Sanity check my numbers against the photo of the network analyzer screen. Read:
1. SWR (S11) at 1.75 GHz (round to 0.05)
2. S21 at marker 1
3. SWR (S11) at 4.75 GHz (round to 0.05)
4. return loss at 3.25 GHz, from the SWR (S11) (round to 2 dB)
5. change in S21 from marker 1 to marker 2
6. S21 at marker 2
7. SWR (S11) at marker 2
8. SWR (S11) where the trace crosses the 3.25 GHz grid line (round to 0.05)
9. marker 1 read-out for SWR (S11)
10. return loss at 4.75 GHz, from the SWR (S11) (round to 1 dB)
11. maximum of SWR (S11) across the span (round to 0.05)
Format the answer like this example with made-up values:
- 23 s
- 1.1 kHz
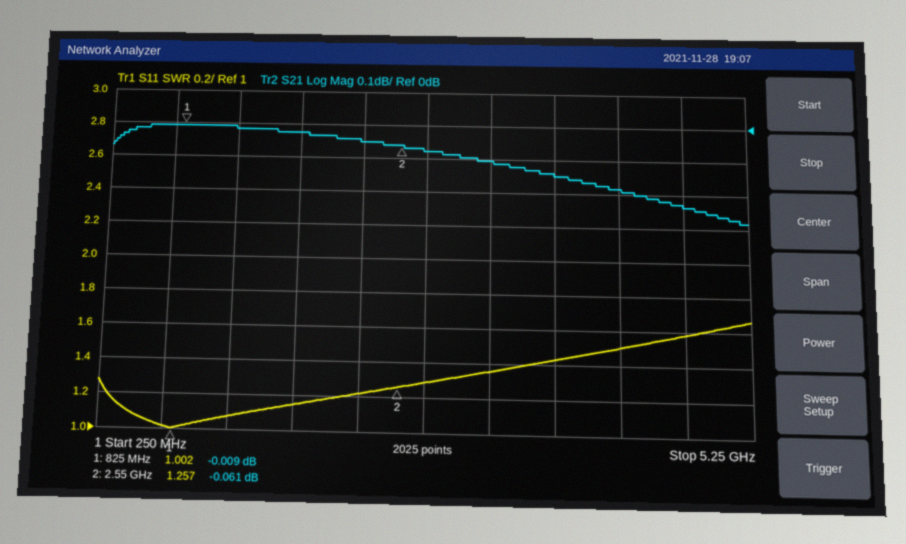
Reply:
- 1.15
- -0.009 dB
- 1.60
- 16 dB
- -0.052 dB
- -0.061 dB
- 1.257
- 1.35
- 1.002
- 13 dB
- 1.65
